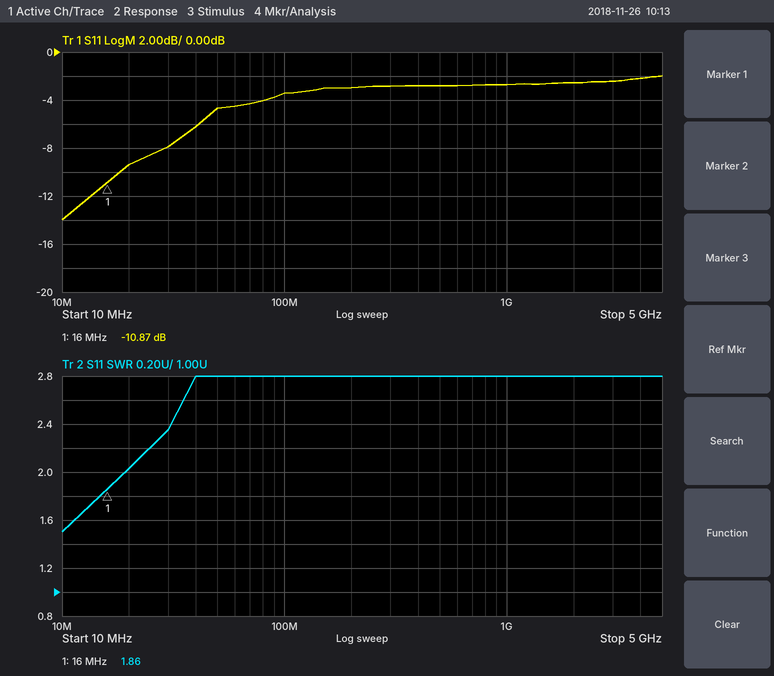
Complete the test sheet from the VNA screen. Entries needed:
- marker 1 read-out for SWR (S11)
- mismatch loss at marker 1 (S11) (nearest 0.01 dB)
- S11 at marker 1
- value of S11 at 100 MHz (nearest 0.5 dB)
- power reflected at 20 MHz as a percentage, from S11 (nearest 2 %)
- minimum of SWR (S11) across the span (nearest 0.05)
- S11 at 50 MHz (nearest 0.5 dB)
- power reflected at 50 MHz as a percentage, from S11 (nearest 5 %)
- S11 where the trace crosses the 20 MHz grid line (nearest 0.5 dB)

1.86
0.37 dB
-10.87 dB
-3.5 dB
12 %
1.50
-4.5 dB
35 %
-9.5 dB
